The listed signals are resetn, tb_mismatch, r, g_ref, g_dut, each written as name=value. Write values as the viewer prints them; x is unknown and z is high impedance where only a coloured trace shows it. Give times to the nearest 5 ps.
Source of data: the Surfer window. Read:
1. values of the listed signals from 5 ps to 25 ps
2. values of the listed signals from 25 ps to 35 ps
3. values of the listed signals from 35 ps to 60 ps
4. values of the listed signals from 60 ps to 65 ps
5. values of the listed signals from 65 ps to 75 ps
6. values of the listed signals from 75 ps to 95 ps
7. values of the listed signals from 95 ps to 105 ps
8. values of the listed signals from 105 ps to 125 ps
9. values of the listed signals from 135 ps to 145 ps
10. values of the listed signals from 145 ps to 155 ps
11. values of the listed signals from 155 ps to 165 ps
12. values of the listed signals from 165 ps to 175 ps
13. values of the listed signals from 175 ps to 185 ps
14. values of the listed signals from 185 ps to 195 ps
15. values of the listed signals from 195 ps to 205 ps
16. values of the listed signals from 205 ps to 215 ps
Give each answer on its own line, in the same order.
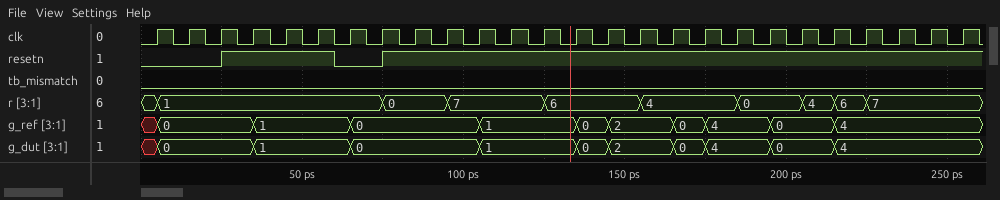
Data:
resetn=0, tb_mismatch=0, r=1, g_ref=0, g_dut=0
resetn=1, tb_mismatch=0, r=1, g_ref=0, g_dut=0
resetn=1, tb_mismatch=0, r=1, g_ref=1, g_dut=1
resetn=0, tb_mismatch=0, r=1, g_ref=1, g_dut=1
resetn=0, tb_mismatch=0, r=1, g_ref=0, g_dut=0
resetn=1, tb_mismatch=0, r=0, g_ref=0, g_dut=0
resetn=1, tb_mismatch=0, r=7, g_ref=0, g_dut=0
resetn=1, tb_mismatch=0, r=7, g_ref=1, g_dut=1
resetn=1, tb_mismatch=0, r=6, g_ref=0, g_dut=0
resetn=1, tb_mismatch=0, r=6, g_ref=2, g_dut=2
resetn=1, tb_mismatch=0, r=4, g_ref=2, g_dut=2
resetn=1, tb_mismatch=0, r=4, g_ref=0, g_dut=0
resetn=1, tb_mismatch=0, r=4, g_ref=4, g_dut=4
resetn=1, tb_mismatch=0, r=0, g_ref=4, g_dut=4
resetn=1, tb_mismatch=0, r=0, g_ref=0, g_dut=0
resetn=1, tb_mismatch=0, r=4, g_ref=0, g_dut=0
